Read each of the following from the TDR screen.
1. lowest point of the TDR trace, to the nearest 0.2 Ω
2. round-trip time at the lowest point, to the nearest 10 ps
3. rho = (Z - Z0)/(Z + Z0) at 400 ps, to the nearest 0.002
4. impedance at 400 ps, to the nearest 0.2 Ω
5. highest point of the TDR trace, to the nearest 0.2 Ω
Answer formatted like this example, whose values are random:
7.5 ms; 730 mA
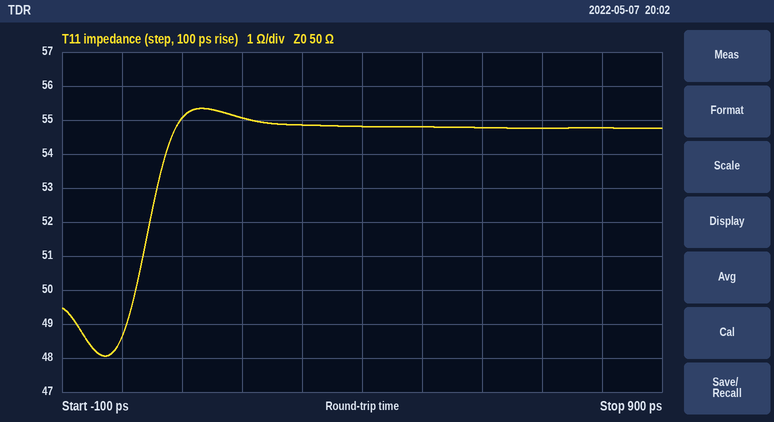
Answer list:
48.0 Ω; -30 ps; +0.046; 54.8 Ω; 55.4 Ω
